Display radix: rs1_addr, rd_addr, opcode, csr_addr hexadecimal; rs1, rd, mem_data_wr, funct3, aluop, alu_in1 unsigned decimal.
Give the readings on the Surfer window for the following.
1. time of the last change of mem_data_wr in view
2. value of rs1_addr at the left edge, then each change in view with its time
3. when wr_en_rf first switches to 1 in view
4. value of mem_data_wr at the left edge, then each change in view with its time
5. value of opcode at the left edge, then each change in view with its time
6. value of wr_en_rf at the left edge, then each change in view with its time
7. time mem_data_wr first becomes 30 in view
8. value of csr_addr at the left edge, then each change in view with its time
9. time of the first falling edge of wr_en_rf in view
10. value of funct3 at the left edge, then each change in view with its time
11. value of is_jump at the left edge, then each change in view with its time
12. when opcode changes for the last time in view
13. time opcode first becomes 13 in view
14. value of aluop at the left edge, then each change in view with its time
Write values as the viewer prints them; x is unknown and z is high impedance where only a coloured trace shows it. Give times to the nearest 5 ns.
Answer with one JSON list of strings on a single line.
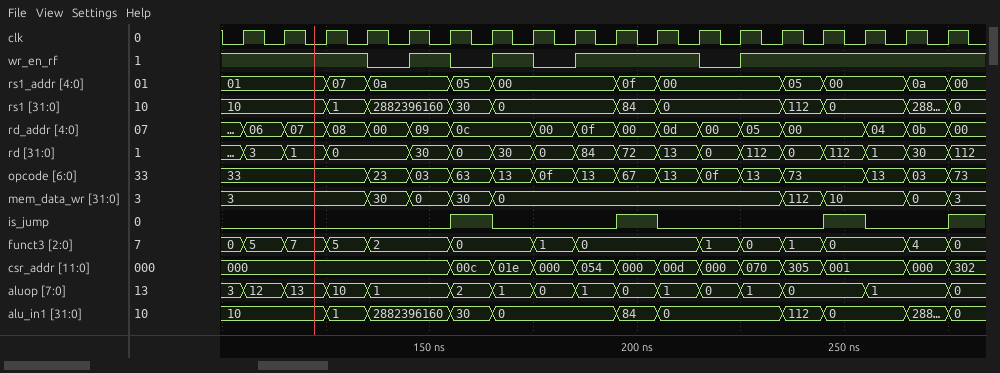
["275 ns", "01, 07 at 125 ns, 0a at 135 ns, 05 at 155 ns, 00 at 165 ns, 0f at 195 ns, 00 at 205 ns, 05 at 235 ns, 00 at 245 ns, 0a at 265 ns, 00 at 275 ns", "145 ns", "3, 30 at 135 ns, 0 at 145 ns, 30 at 155 ns, 0 at 165 ns, 112 at 235 ns, 10 at 245 ns, 0 at 265 ns, 3 at 275 ns", "33, 23 at 135 ns, 03 at 145 ns, 63 at 155 ns, 13 at 165 ns, 0f at 175 ns, 13 at 185 ns, 67 at 195 ns, 13 at 205 ns, 0f at 215 ns, 13 at 225 ns, 73 at 235 ns, 13 at 255 ns, 03 at 265 ns, 73 at 275 ns", "1, 0 at 135 ns, 1 at 145 ns, 0 at 155 ns, 1 at 165 ns, 0 at 175 ns, 1 at 185 ns, 0 at 215 ns, 1 at 225 ns", "135 ns", "000, 00c at 155 ns, 01e at 165 ns, 000 at 175 ns, 054 at 185 ns, 000 at 195 ns, 00d at 205 ns, 000 at 215 ns, 070 at 225 ns, 305 at 235 ns, 001 at 245 ns, 000 at 265 ns, 302 at 275 ns", "135 ns", "0, 5 at 105 ns, 7 at 115 ns, 5 at 125 ns, 2 at 135 ns, 0 at 155 ns, 1 at 175 ns, 0 at 185 ns, 1 at 215 ns, 0 at 225 ns, 1 at 235 ns, 0 at 245 ns, 4 at 265 ns, 0 at 275 ns", "0, 1 at 155 ns, 0 at 165 ns, 1 at 195 ns, 0 at 205 ns, 1 at 245 ns, 0 at 255 ns, 1 at 275 ns", "275 ns", "165 ns", "3, 12 at 105 ns, 13 at 115 ns, 10 at 125 ns, 1 at 135 ns, 2 at 155 ns, 1 at 165 ns, 0 at 175 ns, 1 at 185 ns, 0 at 195 ns, 1 at 205 ns, 0 at 215 ns, 1 at 225 ns, 0 at 235 ns, 1 at 255 ns, 0 at 275 ns"]
